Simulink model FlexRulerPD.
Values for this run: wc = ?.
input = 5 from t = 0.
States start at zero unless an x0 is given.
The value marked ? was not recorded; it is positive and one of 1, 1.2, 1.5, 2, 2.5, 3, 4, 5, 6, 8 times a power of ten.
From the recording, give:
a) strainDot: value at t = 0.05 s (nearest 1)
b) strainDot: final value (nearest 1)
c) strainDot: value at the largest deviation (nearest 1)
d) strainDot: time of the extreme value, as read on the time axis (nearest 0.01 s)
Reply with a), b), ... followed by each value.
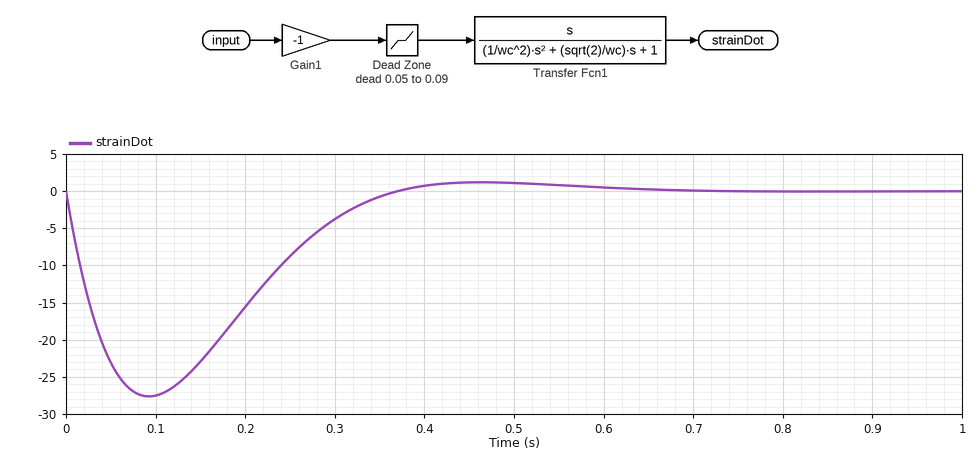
a) -23
b) 0
c) -28
d) 0.09 s
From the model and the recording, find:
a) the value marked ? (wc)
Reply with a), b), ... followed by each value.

a) 12
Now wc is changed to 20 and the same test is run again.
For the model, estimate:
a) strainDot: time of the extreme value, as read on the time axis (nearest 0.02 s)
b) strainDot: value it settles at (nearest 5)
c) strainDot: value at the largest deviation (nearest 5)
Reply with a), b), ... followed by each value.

a) 0.06 s
b) 0
c) -45
